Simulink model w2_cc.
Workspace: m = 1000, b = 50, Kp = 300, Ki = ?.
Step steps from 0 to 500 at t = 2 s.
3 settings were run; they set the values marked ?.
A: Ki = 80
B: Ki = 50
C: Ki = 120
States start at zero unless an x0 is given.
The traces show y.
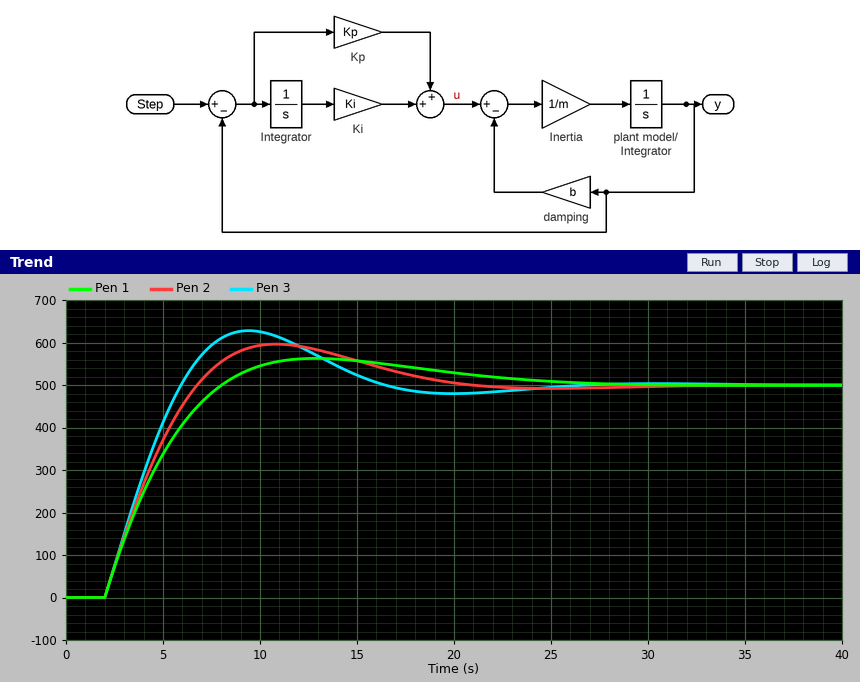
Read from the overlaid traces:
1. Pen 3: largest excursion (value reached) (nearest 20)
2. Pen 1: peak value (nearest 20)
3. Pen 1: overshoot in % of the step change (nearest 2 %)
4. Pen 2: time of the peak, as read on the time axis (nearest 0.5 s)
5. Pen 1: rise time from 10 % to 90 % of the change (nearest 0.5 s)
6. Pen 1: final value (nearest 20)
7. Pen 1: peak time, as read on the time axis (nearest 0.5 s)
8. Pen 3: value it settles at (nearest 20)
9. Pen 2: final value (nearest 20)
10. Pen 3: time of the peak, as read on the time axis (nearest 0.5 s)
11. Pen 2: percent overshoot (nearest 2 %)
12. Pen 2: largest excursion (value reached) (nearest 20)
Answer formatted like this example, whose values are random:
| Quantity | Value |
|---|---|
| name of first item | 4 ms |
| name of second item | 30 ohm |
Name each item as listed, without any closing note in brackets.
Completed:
| Quantity | Value |
|---|---|
| Pen 3: largest excursion (value reached) | 620 |
| Pen 1: peak value | 560 |
| Pen 1: overshoot in % of the step change | 12 % |
| Pen 2: time of the peak, as read on the time axis | 11.0 s |
| Pen 1: rise time from 10 % to 90 % of the change | 4.5 s |
| Pen 1: final value | 500 |
| Pen 1: peak time, as read on the time axis | 13.0 s |
| Pen 3: value it settles at | 500 |
| Pen 2: final value | 500 |
| Pen 3: time of the peak, as read on the time axis | 9.5 s |
| Pen 2: percent overshoot | 20 % |
| Pen 2: largest excursion (value reached) | 600 |
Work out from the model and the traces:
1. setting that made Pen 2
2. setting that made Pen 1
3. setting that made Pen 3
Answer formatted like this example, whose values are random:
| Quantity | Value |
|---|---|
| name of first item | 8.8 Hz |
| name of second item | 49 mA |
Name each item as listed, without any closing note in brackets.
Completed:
| Quantity | Value |
|---|---|
| setting that made Pen 2 | A |
| setting that made Pen 1 | B |
| setting that made Pen 3 | C |
